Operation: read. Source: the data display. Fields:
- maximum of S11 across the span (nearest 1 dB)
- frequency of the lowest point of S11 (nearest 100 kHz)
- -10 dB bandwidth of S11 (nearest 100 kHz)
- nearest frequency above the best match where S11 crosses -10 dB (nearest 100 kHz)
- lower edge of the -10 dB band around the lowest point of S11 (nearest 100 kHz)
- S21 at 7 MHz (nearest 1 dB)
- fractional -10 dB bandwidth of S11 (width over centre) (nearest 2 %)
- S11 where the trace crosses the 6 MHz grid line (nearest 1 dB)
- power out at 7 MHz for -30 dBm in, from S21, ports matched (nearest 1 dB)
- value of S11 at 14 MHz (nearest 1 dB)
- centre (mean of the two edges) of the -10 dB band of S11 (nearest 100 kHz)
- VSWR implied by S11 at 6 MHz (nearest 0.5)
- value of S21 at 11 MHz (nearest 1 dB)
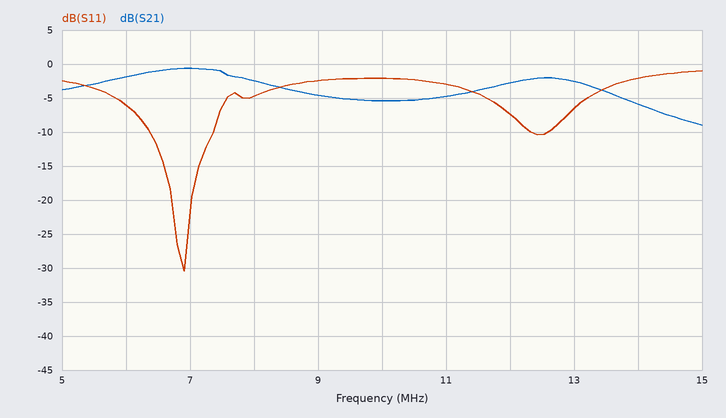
-1 dB
6.9 MHz
1.0 MHz
7.4 MHz
6.4 MHz
-1 dB
14 %
-6 dB
-31 dBm
-2 dB
6.9 MHz
3.0
-5 dB
